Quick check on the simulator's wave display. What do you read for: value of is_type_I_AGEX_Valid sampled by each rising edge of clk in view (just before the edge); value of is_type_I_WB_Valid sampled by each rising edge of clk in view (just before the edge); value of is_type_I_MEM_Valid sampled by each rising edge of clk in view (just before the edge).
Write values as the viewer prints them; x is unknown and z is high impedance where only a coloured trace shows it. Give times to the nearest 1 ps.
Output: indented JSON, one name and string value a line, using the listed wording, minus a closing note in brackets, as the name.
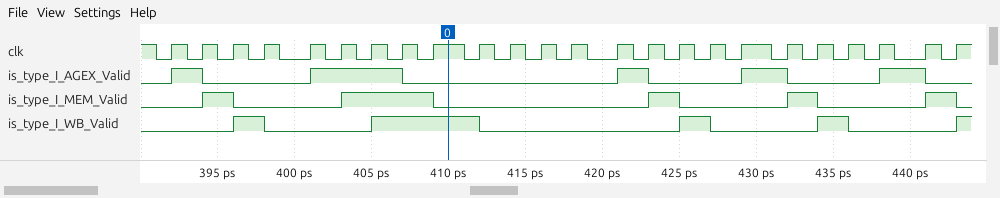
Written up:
{
  "value of is_type_I_AGEX_Valid sampled by each rising edge of clk in view": "0 1 0 0 0 1 1 1 0 0 0 0 0 0 1 0 0 0 1 0 0 0 1 0",
  "value of is_type_I_WB_Valid sampled by each rising edge of clk in view": "0 0 0 1 0 0 0 1 1 1 0 0 0 0 0 0 1 0 0 0 1 0 0 0",
  "value of is_type_I_MEM_Valid sampled by each rising edge of clk in view": "0 0 1 0 0 0 1 1 1 0 0 0 0 0 0 1 0 0 0 1 0 0 0 1"
}
